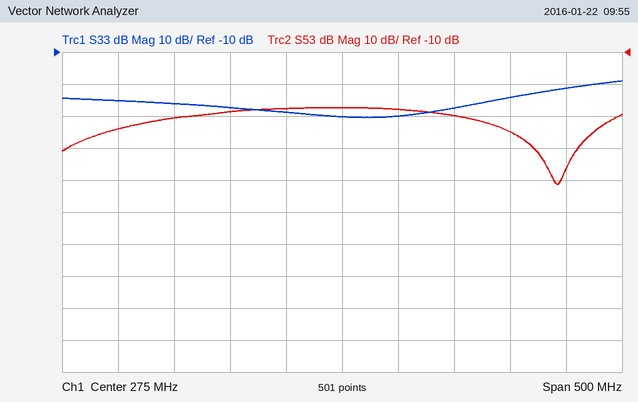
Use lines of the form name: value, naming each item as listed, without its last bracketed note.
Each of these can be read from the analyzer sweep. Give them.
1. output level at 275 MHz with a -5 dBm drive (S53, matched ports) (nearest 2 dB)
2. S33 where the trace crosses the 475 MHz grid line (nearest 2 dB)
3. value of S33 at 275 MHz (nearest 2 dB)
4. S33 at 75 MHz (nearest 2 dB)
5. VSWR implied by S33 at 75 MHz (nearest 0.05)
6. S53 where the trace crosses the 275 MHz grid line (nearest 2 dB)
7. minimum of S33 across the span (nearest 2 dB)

output level at 275 MHz with a -5 dBm drive (S53, matched ports): -32 dBm
S33 where the trace crosses the 475 MHz grid line: -22 dB
value of S33 at 275 MHz: -30 dB
S33 at 75 MHz: -26 dB
VSWR implied by S33 at 75 MHz: 1.10
S53 where the trace crosses the 275 MHz grid line: -28 dB
minimum of S33 across the span: -30 dB
